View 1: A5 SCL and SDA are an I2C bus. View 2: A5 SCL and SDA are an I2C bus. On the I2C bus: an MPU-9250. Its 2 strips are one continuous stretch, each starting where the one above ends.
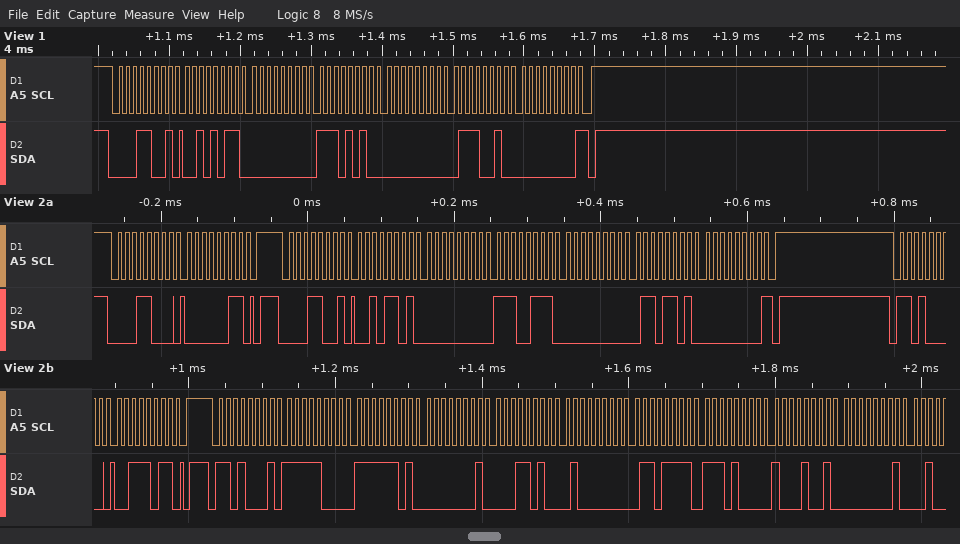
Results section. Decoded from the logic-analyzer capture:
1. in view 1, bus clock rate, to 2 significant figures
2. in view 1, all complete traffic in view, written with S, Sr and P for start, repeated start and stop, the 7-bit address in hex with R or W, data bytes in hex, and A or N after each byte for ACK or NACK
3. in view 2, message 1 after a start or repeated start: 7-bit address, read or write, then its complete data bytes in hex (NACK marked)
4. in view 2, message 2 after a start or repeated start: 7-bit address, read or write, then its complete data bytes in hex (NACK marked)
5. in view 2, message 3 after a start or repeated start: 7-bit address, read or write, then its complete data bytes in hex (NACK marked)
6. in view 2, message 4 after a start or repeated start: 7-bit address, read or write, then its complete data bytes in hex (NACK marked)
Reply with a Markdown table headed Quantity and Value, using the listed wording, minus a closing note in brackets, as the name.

| Quantity | Value |
|---|---|
| in view 1, bus clock rate, to 2 significant figures | 100 kHz |
| in view 1, all complete traffic in view, written with S, Sr and P for start, repeated start and stop, the 7-bit address in hex with R or W, data bytes in hex, and A or N after each byte for ACK or NACK | S 0CR A 2B A 00 A EA A 00 A 72 A 00 N P |
| in view 2, message 1 after a start or repeated start: 7-bit address, read or write, then its complete data bytes in hex | 0x0C write: 03 |
| in view 2, message 2 after a start or repeated start: 7-bit address, read or write, then its complete data bytes in hex | 0x0C read: 2D 00 E7 00 6D 00 NACK |
| in view 2, message 3 after a start or repeated start: 7-bit address, read or write, then its complete data bytes in hex | 0x68 write: 3B |
| in view 2, message 4 after a start or repeated start: 7-bit address, read or write, then its complete data bytes in hex | 0x68 read: F8 FD 01 1A 40 6F E8 89 01 |
